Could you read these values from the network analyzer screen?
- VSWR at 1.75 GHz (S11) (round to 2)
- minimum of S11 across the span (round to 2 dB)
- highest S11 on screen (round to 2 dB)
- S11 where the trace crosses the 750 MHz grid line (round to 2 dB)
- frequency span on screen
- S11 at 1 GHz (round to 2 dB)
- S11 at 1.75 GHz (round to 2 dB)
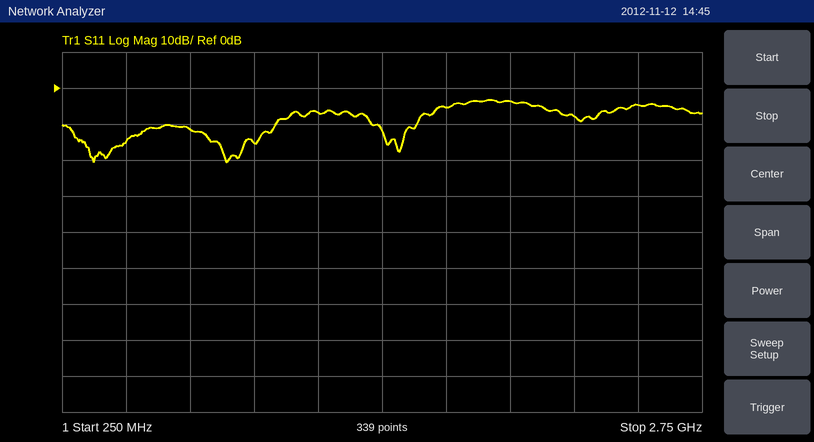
4
-20 dB
-4 dB
-12 dB
2.5 GHz
-16 dB
-6 dB
